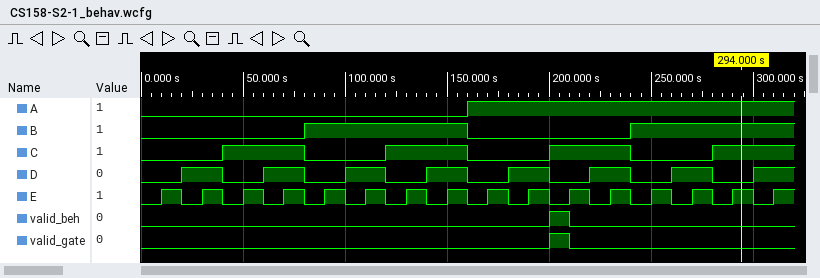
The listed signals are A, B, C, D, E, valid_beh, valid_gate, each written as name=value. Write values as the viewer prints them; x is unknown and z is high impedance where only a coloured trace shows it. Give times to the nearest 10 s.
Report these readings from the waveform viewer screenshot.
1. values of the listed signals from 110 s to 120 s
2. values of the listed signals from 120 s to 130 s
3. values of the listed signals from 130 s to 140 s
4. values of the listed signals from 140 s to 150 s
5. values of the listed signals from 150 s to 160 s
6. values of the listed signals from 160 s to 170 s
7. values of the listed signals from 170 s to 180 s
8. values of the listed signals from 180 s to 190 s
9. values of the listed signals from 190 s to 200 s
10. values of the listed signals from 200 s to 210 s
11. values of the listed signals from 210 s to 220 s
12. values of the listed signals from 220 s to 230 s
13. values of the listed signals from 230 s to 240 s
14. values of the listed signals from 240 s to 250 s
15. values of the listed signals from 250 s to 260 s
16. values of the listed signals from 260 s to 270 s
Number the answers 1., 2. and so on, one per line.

1. A=0, B=1, C=0, D=1, E=1, valid_beh=0, valid_gate=0
2. A=0, B=1, C=1, D=0, E=0, valid_beh=0, valid_gate=0
3. A=0, B=1, C=1, D=0, E=1, valid_beh=0, valid_gate=0
4. A=0, B=1, C=1, D=1, E=0, valid_beh=0, valid_gate=0
5. A=0, B=1, C=1, D=1, E=1, valid_beh=0, valid_gate=0
6. A=1, B=0, C=0, D=0, E=0, valid_beh=0, valid_gate=0
7. A=1, B=0, C=0, D=0, E=1, valid_beh=0, valid_gate=0
8. A=1, B=0, C=0, D=1, E=0, valid_beh=0, valid_gate=0
9. A=1, B=0, C=0, D=1, E=1, valid_beh=0, valid_gate=0
10. A=1, B=0, C=1, D=0, E=0, valid_beh=1, valid_gate=1
11. A=1, B=0, C=1, D=0, E=1, valid_beh=0, valid_gate=0
12. A=1, B=0, C=1, D=1, E=0, valid_beh=0, valid_gate=0
13. A=1, B=0, C=1, D=1, E=1, valid_beh=0, valid_gate=0
14. A=1, B=1, C=0, D=0, E=0, valid_beh=0, valid_gate=0
15. A=1, B=1, C=0, D=0, E=1, valid_beh=0, valid_gate=0
16. A=1, B=1, C=0, D=1, E=0, valid_beh=0, valid_gate=0
